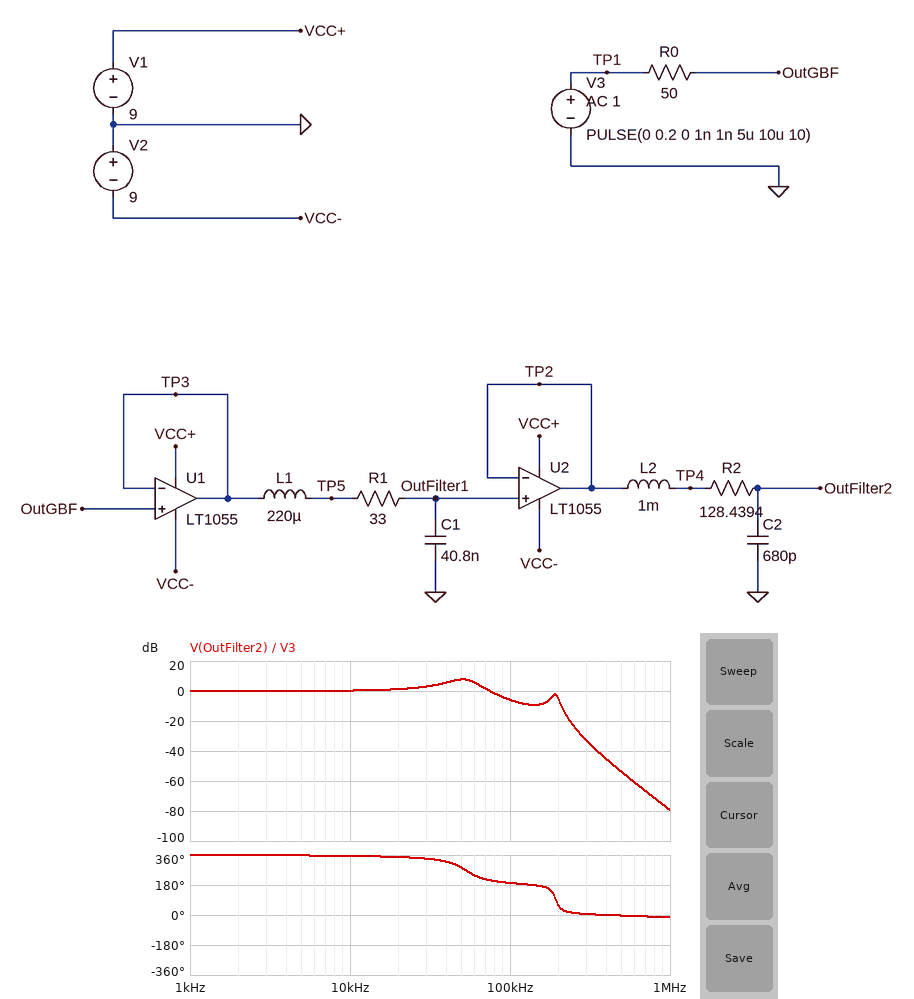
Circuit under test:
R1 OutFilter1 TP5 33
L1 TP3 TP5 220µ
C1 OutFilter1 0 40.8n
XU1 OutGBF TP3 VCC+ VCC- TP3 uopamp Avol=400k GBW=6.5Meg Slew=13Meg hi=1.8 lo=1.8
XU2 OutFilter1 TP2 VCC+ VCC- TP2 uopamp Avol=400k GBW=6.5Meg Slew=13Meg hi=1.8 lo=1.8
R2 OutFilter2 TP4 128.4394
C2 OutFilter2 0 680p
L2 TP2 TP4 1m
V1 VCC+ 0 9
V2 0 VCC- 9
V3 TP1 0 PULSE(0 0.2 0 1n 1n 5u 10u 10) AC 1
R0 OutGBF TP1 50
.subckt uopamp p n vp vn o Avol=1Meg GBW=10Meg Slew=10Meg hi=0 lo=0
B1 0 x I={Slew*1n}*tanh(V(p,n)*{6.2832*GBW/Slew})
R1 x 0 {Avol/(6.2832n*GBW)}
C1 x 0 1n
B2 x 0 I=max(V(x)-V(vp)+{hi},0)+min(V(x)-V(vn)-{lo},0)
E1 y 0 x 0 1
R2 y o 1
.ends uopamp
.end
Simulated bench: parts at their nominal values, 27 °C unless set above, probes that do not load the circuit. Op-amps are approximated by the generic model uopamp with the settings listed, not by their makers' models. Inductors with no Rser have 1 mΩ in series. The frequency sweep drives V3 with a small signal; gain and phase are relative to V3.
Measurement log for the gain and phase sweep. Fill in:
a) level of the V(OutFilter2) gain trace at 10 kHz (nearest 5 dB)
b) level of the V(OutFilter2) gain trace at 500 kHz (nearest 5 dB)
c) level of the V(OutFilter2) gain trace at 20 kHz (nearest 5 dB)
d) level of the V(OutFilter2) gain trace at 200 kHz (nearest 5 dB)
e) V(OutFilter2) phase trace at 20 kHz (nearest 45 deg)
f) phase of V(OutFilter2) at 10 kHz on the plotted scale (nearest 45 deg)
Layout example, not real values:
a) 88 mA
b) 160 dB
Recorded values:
a) 0 dB
b) -55 dB
c) 0 dB
d) -5 dB
e) 360 deg
f) 360 deg
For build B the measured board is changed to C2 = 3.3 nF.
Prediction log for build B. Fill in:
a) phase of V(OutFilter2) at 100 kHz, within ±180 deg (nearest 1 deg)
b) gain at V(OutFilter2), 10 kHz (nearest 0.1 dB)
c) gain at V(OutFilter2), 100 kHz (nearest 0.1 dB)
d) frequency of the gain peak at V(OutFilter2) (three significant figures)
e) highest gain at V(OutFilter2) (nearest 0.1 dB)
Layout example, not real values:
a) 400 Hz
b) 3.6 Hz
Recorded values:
a) 58 deg
b) 0.4 dB
c) -0.7 dB
d) 53.3 kHz
e) 10.7 dB
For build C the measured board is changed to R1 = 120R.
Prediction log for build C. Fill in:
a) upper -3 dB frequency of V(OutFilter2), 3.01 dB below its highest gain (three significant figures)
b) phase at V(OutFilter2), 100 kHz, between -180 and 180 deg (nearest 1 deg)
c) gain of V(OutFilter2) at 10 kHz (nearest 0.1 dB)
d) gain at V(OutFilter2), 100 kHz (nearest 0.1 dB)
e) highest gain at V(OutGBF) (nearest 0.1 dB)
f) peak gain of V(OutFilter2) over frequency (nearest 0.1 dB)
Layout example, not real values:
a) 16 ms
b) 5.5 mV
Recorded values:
a) 48.8 kHz
b) -136 deg
c) -0.1 dB
d) -9.3 dB
e) 0 dB
f) 0 dB
